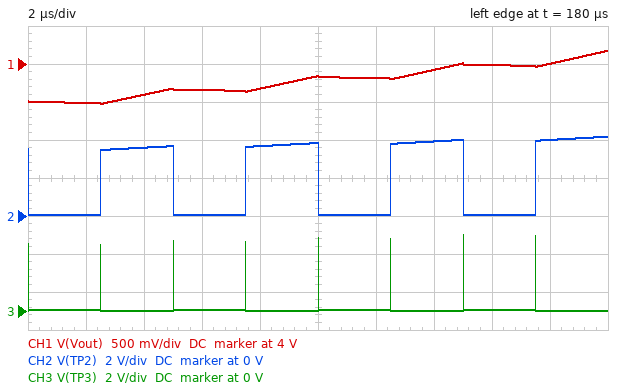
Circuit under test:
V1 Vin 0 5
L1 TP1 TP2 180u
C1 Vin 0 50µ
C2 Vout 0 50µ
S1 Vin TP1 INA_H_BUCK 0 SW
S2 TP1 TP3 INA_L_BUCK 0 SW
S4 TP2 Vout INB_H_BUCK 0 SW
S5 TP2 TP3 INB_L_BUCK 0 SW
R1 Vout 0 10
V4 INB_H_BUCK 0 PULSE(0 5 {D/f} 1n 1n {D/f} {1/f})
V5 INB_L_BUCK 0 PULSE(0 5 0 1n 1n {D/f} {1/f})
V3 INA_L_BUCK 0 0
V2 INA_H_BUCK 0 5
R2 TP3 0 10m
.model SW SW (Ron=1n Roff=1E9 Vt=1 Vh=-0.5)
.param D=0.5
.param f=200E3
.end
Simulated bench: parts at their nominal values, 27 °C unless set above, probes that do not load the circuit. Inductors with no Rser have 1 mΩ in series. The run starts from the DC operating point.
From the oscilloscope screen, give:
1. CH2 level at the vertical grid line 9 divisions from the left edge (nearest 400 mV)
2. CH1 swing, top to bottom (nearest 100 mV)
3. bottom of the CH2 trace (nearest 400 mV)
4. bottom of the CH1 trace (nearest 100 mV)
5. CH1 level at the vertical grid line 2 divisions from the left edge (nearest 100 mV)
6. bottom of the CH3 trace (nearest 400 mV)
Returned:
4.0 V
700 mV
0 V
3.5 V
3.6 V
0 V
